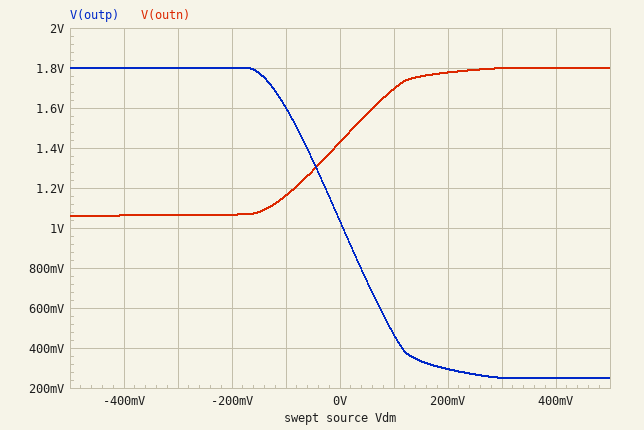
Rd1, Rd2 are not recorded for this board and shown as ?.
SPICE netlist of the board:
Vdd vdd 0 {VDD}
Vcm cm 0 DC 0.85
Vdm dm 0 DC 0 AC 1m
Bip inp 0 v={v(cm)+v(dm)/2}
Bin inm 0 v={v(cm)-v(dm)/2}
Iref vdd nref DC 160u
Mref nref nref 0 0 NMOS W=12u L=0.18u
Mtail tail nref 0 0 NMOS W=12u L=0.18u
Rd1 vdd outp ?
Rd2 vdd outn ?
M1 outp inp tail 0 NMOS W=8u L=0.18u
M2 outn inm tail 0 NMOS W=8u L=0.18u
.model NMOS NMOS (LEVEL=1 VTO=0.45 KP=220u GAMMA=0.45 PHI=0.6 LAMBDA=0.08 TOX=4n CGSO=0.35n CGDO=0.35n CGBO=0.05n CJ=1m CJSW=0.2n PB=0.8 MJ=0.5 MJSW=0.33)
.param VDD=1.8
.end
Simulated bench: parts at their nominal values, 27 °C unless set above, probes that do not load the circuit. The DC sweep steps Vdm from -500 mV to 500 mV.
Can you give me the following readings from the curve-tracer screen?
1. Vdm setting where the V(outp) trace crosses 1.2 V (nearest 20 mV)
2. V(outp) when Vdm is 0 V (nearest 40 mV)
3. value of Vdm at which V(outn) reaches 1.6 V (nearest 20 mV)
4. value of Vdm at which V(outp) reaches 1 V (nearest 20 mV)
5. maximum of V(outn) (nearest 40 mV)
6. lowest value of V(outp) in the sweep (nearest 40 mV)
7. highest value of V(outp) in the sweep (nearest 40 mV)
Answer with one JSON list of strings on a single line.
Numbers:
["-20 mV", "1.04 V", "60 mV", "0 V", "1.80 V", "240 mV", "1.80 V"]
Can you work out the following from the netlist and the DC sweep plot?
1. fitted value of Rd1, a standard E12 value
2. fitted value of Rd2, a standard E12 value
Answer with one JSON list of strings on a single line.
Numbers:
["10 kΩ", "4.7 kΩ"]
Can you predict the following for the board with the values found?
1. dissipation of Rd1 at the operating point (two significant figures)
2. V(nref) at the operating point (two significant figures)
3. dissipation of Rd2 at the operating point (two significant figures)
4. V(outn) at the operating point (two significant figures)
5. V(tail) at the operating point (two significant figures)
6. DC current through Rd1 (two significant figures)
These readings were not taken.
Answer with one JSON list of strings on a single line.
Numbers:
["59 µW", "590 mV", "29 µW", "1.4 V", "220 mV", "77 µA"]
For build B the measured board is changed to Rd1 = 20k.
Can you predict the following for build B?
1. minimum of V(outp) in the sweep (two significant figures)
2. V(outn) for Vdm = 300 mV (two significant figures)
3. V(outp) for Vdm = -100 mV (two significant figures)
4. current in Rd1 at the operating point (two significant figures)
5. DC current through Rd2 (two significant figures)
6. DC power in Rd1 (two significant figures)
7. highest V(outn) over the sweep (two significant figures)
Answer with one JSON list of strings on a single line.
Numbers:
["82 mV", "1.5 V", "1.4 V", "74 µA", "82 µA", "110 µW", "1.7 V"]
